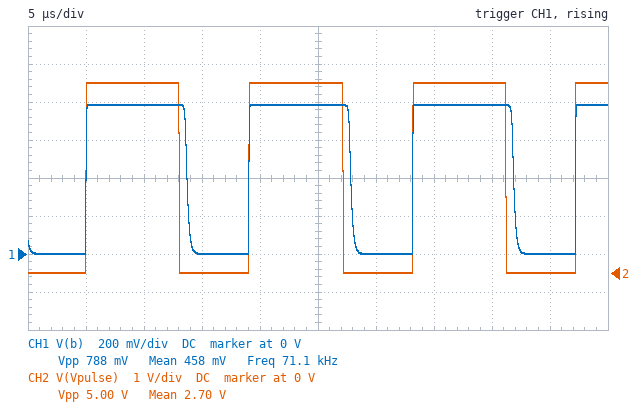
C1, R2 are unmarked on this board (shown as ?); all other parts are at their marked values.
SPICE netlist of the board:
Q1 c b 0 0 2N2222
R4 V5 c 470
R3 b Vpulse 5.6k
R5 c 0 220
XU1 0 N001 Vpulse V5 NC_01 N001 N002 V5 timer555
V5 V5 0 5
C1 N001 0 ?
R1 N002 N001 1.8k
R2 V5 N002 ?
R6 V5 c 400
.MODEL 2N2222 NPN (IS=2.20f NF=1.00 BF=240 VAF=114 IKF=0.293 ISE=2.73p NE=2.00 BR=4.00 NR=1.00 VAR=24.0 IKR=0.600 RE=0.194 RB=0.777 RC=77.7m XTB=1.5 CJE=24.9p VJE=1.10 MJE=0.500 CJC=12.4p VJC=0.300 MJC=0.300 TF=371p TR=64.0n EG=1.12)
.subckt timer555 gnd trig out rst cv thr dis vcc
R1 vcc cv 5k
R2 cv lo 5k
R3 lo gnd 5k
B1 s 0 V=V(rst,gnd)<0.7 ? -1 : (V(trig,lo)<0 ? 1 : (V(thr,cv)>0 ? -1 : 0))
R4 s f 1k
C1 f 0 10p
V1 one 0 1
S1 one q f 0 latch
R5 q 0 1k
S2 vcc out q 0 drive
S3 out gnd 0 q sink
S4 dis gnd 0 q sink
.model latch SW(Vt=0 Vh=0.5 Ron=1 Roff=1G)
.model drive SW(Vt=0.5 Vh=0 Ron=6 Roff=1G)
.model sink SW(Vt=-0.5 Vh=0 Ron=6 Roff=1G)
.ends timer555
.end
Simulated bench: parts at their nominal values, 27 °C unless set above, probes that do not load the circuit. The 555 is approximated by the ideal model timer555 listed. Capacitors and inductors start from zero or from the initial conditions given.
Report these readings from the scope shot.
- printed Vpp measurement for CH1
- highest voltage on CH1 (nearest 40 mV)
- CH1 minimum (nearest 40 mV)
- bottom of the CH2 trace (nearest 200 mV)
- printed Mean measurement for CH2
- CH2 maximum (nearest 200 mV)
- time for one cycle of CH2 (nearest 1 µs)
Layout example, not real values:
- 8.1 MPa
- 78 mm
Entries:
- 788 mV
- 800 mV
- 0 V
- 0 V
- 2.70 V
- 5.0 V
- 14 µs
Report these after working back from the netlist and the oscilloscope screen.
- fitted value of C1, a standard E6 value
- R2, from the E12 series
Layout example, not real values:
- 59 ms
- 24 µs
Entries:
- 4.7 nF
- 680 Ω
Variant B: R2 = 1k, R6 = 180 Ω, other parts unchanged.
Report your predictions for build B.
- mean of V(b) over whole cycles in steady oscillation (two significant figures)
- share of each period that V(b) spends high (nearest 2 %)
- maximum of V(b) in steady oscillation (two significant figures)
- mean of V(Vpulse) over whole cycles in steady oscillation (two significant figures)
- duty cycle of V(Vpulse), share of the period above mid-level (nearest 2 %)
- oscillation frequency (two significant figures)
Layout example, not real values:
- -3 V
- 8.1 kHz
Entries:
- 520 mV
- 64 %
- 800 mV
- 3.0 V
- 60 %
- 66 kHz
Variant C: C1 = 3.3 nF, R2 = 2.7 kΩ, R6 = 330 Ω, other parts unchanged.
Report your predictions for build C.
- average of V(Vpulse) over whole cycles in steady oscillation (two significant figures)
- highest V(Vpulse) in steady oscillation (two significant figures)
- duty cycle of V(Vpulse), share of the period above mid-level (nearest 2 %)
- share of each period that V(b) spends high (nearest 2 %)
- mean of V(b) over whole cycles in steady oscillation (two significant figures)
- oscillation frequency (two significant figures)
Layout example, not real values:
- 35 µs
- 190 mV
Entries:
- 3.6 V
- 5.0 V
- 72 %
- 76 %
- 600 mV
- 69 kHz
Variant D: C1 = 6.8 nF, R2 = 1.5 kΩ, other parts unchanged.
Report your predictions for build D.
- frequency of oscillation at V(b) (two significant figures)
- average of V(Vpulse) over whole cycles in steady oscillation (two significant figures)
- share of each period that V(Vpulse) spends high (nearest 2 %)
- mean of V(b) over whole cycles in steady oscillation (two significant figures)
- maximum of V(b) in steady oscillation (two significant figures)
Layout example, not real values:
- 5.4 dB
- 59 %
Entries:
- 41 kHz
- 3.2 V
- 64 %
- 530 mV
- 790 mV
